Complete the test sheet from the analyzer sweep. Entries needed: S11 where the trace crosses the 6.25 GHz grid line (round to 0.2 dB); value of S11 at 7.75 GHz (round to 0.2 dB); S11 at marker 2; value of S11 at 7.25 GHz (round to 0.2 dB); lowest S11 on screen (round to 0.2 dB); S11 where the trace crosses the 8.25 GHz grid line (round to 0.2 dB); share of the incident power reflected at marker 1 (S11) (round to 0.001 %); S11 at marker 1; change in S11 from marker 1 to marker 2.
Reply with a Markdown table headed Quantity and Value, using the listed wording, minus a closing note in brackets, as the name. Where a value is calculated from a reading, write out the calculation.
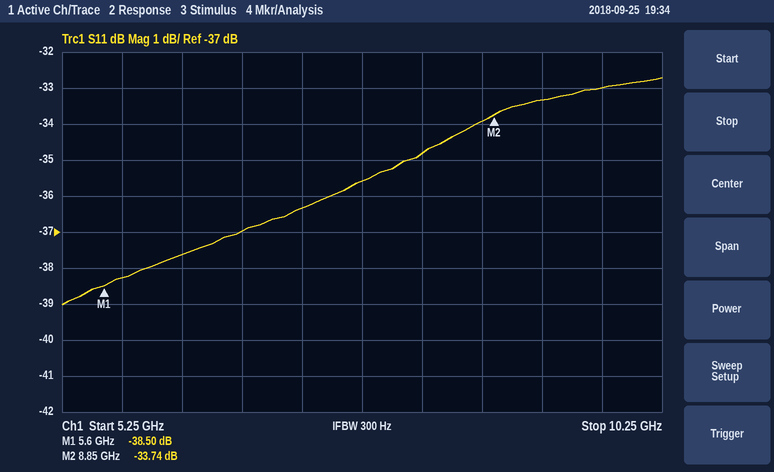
| Quantity | Value |
|---|---|
| S11 where the trace crosses the 6.25 GHz grid line | -37.6 dB |
| value of S11 at 7.75 GHz | -35.6 dB |
| S11 at marker 2 | -33.74 dB |
| value of S11 at 7.25 GHz | -36.4 dB |
| lowest S11 on screen | -39.0 dB |
| S11 where the trace crosses the 8.25 GHz grid line | -34.8 dB |
| share of the incident power reflected at marker 1 (S11) | 10^(-38.5/10) ≈ 0.014 % |
| S11 at marker 1 | -38.50 dB |
| change in S11 from marker 1 to marker 2 | -33.74 − (-38.5) = 4.76 dB |
